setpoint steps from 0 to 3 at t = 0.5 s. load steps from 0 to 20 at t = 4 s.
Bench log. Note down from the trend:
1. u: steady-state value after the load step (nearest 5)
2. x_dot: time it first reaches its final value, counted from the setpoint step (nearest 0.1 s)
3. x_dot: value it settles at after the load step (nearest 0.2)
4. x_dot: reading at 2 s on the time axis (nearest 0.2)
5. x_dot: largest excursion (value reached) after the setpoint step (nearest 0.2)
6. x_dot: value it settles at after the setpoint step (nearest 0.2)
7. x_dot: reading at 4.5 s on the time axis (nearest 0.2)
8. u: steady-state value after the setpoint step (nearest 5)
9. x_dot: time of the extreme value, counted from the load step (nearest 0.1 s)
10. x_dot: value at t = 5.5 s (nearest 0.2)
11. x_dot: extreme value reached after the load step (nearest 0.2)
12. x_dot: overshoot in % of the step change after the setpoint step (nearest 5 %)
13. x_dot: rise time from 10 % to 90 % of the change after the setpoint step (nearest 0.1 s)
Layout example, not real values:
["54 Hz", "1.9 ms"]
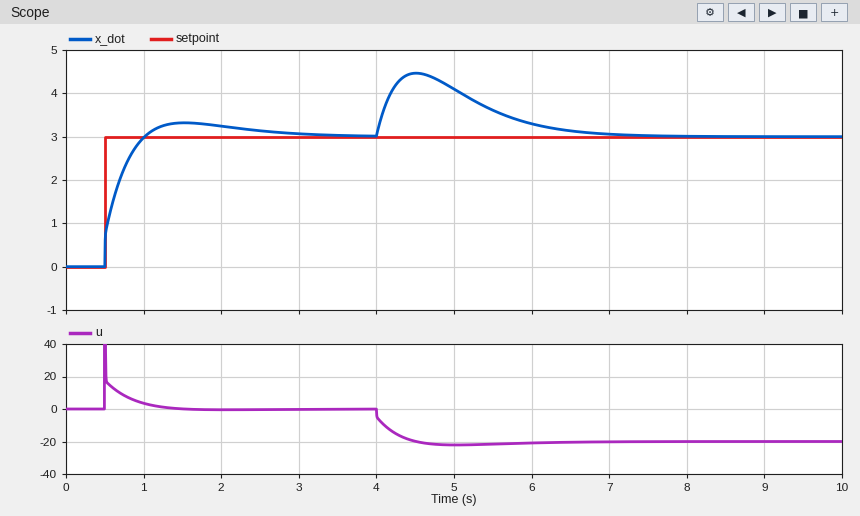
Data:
["-20", "0.5 s", "3.0", "3.2", "3.4", "3.0", "4.4", "0", "0.5 s", "3.6", "4.4", "10 %", "0.4 s"]
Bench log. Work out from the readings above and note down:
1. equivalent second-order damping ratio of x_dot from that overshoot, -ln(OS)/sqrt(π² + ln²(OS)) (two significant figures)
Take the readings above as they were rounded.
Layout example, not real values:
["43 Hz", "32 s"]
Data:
["0.59"]
